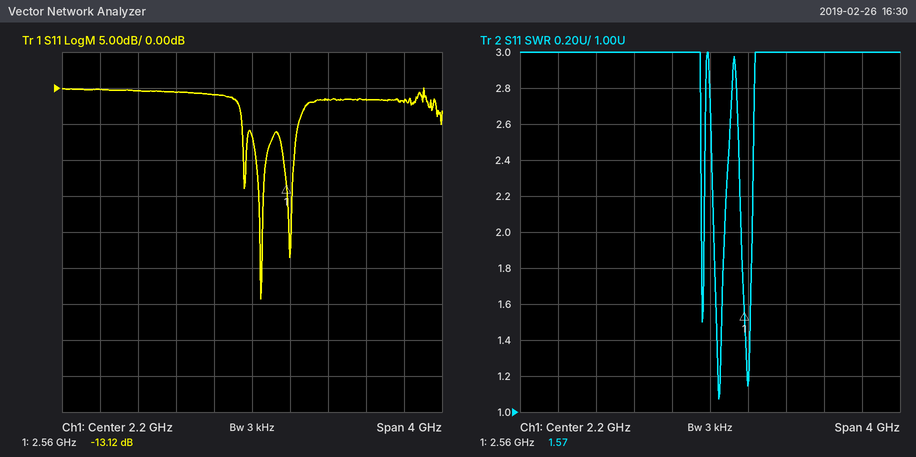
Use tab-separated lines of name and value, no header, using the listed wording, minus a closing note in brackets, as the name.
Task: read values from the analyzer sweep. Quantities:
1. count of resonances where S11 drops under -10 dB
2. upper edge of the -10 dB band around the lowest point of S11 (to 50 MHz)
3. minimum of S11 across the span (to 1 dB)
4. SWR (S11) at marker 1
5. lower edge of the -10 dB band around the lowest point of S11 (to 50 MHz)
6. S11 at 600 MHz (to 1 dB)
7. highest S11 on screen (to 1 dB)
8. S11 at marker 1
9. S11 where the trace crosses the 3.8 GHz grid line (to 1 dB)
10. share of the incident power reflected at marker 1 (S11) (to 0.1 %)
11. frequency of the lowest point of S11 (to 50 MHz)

count of resonances where S11 drops under -10 dB	3
upper edge of the -10 dB band around the lowest point of S11	2.35 GHz
minimum of S11 across the span	-29 dB
SWR (S11) at marker 1	1.57
lower edge of the -10 dB band around the lowest point of S11	2.25 GHz
S11 at 600 MHz	0 dB
highest S11 on screen	0 dB
S11 at marker 1	-13.12 dB
S11 where the trace crosses the 3.8 GHz grid line	-2 dB
share of the incident power reflected at marker 1 (S11)	4.9 %
frequency of the lowest point of S11	2.30 GHz
